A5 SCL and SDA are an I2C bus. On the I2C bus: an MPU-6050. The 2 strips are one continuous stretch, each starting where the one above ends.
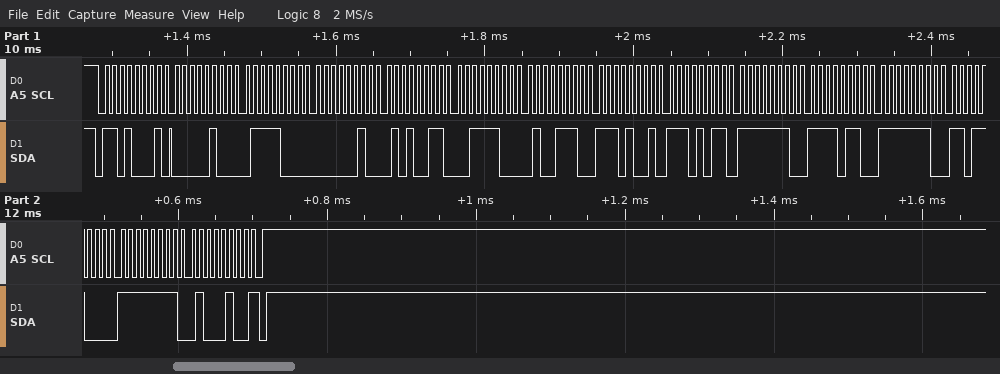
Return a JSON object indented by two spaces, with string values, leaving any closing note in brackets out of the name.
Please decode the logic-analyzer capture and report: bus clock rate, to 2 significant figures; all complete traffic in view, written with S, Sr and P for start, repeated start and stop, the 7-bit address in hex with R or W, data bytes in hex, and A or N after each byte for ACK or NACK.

{
  "bus clock rate, to 2 significant figures": "100 kHz",
  "all complete traffic in view, written with S, Sr and P for start, repeated start and stop, the 7-bit address in hex with R or W, data bytes in hex, and A or N after each byte for ACK or NACK": "S 68R A 04 A 78 A 02 A 53 A 3C A 4E A E9 A EB A FE A F6 A FE A D8 A FF A 44 N P"
}
